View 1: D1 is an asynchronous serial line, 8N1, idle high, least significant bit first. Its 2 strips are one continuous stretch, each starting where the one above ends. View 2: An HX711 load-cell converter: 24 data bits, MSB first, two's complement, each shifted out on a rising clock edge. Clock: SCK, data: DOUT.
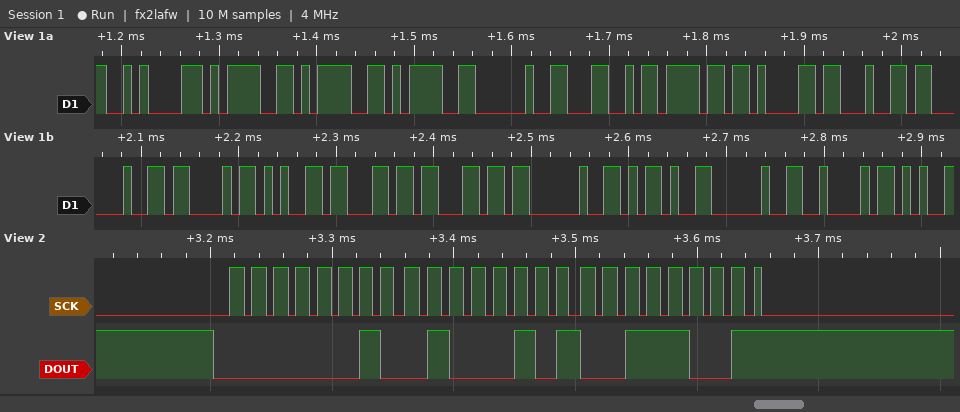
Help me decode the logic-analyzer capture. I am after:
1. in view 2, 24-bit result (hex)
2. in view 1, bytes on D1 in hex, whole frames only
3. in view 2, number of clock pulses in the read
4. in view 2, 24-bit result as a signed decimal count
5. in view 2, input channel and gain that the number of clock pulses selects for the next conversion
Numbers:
0x024539
0A 3D 3D 3D 20 4C 6F 61 64 20 43 65 6C 6C 20 2D 20 42
25
148793
channel A, gain 128
